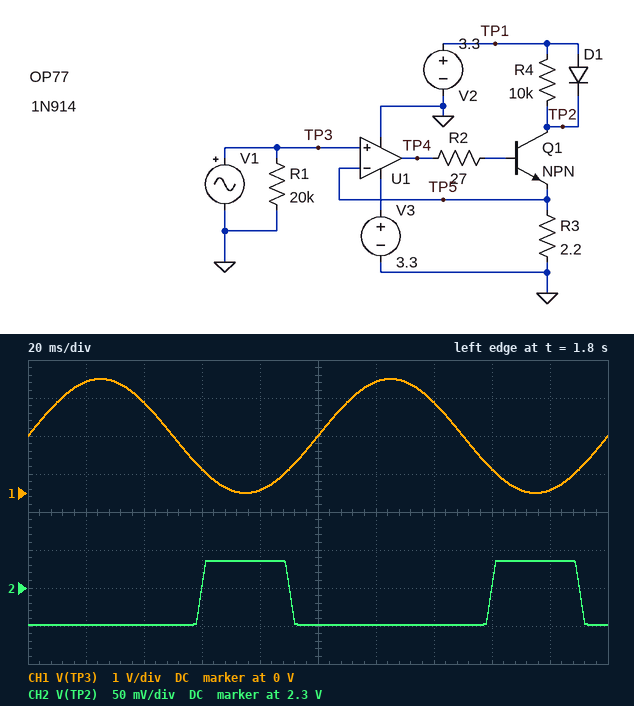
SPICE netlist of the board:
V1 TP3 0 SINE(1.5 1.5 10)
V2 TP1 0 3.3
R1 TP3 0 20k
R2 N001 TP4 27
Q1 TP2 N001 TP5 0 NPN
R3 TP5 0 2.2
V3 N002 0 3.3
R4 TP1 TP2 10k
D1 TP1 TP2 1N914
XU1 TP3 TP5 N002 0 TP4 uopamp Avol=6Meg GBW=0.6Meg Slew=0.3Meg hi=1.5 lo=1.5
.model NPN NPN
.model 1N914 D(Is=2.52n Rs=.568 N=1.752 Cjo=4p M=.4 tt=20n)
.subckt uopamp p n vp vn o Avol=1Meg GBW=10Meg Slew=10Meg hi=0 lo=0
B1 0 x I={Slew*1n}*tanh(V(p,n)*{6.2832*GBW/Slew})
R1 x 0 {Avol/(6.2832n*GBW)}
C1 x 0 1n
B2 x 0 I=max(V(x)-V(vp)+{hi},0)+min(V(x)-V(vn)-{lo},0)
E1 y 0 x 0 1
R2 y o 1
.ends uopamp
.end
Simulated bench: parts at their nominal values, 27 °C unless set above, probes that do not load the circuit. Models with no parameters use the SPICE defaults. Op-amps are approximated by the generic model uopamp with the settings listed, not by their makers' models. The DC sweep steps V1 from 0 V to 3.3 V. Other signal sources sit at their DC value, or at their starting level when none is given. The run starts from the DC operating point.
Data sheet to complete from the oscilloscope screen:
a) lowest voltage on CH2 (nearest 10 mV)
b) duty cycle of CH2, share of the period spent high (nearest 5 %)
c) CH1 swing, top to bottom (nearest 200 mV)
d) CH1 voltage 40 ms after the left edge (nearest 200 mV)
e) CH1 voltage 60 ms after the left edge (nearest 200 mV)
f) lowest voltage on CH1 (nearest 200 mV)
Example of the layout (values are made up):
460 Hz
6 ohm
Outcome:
2.25 V
30 %
3.0 V
2.4 V
600 mV
0 V
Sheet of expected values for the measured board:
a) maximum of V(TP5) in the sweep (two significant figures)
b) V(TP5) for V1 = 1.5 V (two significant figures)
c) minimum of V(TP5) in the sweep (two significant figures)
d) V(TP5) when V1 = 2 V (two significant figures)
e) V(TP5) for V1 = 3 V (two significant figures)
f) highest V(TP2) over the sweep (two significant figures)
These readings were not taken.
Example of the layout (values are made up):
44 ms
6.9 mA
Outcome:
780 mV
780 mV
520 mV
780 mV
780 mV
2.3 V
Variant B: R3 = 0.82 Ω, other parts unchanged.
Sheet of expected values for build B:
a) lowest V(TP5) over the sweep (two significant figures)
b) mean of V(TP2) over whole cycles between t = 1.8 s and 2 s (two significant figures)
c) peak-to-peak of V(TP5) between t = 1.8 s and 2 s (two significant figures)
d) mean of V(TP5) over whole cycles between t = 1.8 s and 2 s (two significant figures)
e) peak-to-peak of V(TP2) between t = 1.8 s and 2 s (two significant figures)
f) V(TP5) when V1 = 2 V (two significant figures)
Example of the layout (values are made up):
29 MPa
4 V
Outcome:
420 mV
2.0 V
220 mV
580 mV
170 mV
640 mV
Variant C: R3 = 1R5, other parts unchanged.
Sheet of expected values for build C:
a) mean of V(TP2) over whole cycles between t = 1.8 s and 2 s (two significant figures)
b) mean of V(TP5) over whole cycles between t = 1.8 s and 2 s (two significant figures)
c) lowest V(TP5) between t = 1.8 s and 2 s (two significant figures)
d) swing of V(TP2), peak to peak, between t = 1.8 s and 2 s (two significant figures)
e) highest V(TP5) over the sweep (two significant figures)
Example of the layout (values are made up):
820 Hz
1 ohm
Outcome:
2.2 V
660 mV
490 mV
110 mV
730 mV
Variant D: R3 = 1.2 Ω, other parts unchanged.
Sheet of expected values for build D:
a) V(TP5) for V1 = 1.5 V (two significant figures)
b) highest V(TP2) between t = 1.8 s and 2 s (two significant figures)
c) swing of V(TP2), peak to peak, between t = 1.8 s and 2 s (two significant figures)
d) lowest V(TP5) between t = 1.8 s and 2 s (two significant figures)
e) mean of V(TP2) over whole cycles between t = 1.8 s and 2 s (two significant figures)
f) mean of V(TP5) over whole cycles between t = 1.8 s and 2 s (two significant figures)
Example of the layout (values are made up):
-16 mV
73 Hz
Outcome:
700 mV
2.2 V
130 mV
460 mV
2.1 V
630 mV
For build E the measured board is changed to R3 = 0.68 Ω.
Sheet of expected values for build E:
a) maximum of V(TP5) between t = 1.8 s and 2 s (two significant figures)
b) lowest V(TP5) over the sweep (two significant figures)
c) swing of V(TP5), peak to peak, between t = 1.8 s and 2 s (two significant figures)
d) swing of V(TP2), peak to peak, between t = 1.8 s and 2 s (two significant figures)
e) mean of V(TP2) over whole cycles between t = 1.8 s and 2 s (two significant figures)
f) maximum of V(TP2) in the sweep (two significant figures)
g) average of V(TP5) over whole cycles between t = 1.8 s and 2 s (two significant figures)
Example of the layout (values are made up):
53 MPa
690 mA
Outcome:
600 mV
400 mV
210 mV
190 mV
2.0 V
2.1 V
550 mV
